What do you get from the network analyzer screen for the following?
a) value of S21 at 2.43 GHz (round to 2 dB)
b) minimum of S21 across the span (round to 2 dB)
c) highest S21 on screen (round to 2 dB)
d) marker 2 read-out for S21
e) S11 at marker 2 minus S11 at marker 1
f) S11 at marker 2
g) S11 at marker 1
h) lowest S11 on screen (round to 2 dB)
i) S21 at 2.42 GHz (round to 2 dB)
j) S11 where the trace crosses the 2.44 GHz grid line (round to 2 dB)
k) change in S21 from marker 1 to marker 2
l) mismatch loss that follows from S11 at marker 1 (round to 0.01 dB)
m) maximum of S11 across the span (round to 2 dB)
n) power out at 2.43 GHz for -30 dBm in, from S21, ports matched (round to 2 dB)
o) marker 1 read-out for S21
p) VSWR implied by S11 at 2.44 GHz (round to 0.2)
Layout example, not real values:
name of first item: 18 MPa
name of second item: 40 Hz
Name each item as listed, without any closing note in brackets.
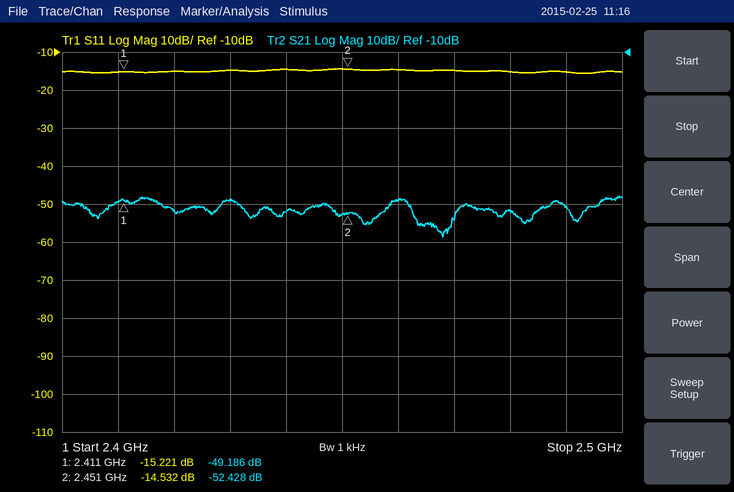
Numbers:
value of S21 at 2.43 GHz: -48 dB
minimum of S21 across the span: -58 dB
highest S21 on screen: -48 dB
marker 2 read-out for S21: -52.428 dB
S11 at marker 2 minus S11 at marker 1: 0.689 dB
S11 at marker 2: -14.532 dB
S11 at marker 1: -15.221 dB
lowest S11 on screen: -16 dB
S21 at 2.42 GHz: -52 dB
S11 where the trace crosses the 2.44 GHz grid line: -14 dB
change in S21 from marker 1 to marker 2: -3.242 dB
mismatch loss that follows from S11 at marker 1: 0.13 dB
maximum of S11 across the span: -14 dB
power out at 2.43 GHz for -30 dBm in, from S21, ports matched: -78 dBm
marker 1 read-out for S21: -49.186 dB
VSWR implied by S11 at 2.44 GHz: 1.4
